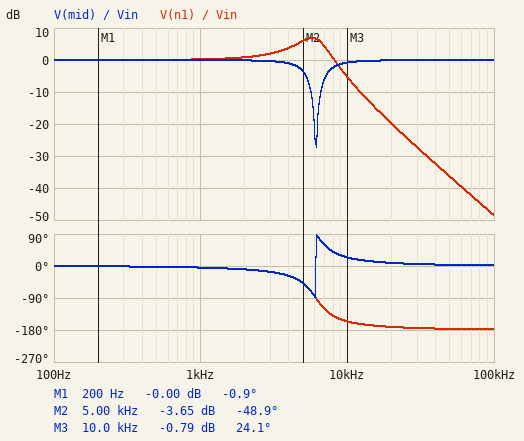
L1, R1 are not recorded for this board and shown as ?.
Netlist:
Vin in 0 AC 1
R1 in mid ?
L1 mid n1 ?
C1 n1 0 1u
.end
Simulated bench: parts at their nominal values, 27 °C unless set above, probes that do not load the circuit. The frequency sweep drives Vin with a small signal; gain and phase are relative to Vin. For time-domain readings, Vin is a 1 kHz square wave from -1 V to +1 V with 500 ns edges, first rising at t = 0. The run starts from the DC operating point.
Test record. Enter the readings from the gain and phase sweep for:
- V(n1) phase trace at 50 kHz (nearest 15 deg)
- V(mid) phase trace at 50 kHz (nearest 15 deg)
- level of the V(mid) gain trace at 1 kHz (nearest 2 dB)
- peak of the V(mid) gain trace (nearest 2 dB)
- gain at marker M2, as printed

-180 deg
0 deg
0 dB
0 dB
-3.65 dB
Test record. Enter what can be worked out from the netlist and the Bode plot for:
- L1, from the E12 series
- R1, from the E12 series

680 µH
12 Ω
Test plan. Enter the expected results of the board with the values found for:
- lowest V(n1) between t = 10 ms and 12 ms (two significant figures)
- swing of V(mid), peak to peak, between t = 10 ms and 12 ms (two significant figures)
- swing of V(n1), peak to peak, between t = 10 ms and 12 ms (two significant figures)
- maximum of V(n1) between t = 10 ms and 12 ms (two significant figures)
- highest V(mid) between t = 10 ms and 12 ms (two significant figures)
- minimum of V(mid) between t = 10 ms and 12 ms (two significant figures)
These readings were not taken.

-1.9 V
2.6 V
3.9 V
1.9 V
1.3 V
-1.3 V
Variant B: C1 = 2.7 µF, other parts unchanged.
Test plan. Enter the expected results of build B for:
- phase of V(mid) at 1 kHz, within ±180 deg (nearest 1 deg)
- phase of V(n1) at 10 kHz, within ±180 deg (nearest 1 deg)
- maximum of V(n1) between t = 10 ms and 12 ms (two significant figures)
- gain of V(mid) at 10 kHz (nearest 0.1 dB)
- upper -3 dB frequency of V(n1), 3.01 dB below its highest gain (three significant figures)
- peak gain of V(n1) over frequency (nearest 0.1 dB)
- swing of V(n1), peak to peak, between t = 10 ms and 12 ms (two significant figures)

-12 deg
-162 deg
1.6 V
-0.4 dB
4.42 kHz
3.1 dB
3.1 V
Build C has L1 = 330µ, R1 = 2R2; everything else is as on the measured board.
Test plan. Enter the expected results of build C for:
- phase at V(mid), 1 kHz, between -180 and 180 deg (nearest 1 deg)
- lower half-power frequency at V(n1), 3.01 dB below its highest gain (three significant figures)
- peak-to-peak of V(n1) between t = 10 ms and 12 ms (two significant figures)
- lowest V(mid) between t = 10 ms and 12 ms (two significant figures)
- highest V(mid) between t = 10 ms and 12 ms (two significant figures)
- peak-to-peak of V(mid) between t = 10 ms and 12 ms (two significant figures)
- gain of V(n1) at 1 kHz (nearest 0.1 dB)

-1 deg
8.18 kHz
5.7 V
-1.2 V
1.2 V
2.4 V
0.1 dB
